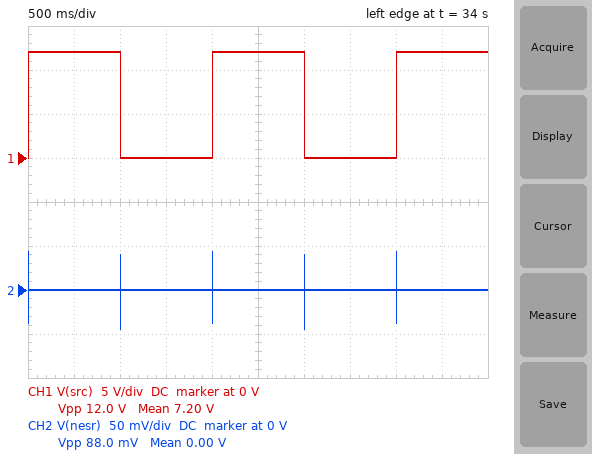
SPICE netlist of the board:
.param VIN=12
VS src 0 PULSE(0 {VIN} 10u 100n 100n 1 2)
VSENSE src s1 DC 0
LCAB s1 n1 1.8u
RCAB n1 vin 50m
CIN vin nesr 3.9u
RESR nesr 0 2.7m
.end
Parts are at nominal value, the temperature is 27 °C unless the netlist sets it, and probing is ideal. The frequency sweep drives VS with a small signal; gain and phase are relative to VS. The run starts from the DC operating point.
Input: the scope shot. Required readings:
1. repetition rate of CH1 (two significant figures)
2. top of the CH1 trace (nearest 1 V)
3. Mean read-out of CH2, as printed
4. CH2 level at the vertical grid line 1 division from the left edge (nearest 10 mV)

500 mHz
12 V
0.00 V
0 V
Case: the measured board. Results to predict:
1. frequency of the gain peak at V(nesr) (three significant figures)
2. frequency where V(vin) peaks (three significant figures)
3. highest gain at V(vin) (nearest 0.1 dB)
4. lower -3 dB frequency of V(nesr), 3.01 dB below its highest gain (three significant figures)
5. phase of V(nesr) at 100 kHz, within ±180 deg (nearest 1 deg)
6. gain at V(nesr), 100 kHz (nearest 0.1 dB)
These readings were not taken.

60.1 kHz
60.0 kHz
22.2 dB
57.8 kHz
-86 deg
-48.6 dB
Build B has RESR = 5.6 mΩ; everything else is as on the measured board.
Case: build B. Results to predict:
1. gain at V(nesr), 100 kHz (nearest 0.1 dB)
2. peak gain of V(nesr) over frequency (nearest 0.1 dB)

-42.2 dB
-19.9 dB
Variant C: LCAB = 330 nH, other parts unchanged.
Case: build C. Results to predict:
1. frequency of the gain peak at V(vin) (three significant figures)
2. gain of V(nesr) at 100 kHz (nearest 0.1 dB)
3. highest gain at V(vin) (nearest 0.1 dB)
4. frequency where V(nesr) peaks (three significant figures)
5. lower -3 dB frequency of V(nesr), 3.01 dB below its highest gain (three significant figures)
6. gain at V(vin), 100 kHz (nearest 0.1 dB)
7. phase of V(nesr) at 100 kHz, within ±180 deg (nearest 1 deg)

139 kHz
-37.7 dB
14.9 dB
140 kHz
128 kHz
5.9 dB
75 deg
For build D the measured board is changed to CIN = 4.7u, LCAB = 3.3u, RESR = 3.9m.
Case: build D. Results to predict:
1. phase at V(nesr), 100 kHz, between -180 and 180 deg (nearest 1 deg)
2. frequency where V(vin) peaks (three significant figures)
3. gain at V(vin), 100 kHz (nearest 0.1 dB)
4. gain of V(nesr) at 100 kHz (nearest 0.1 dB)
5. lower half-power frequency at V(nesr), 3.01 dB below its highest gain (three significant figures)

-88 deg
40.4 kHz
-14.2 dB
-53.0 dB
39.1 kHz
